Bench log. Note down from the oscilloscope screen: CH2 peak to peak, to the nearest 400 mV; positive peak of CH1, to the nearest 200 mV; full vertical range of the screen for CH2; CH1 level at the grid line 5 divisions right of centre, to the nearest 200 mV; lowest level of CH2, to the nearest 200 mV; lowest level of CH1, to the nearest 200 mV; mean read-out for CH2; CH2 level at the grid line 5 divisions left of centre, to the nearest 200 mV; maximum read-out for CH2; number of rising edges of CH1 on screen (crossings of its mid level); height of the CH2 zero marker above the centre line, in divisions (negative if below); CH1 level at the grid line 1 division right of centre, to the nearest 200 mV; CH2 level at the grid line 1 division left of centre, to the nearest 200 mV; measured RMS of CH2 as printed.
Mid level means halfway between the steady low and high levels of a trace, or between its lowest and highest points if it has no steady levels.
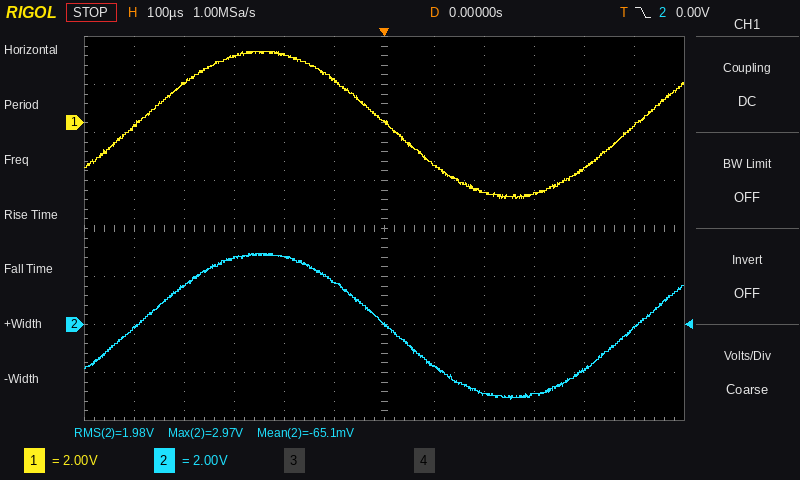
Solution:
6.0 V
3.0 V
16 V
-200 mV
-3.2 V
-3.2 V
-65.1 mV
-200 mV
2.97 V
2
-2.0 div
-1.8 V
1.8 V
1.98 V
